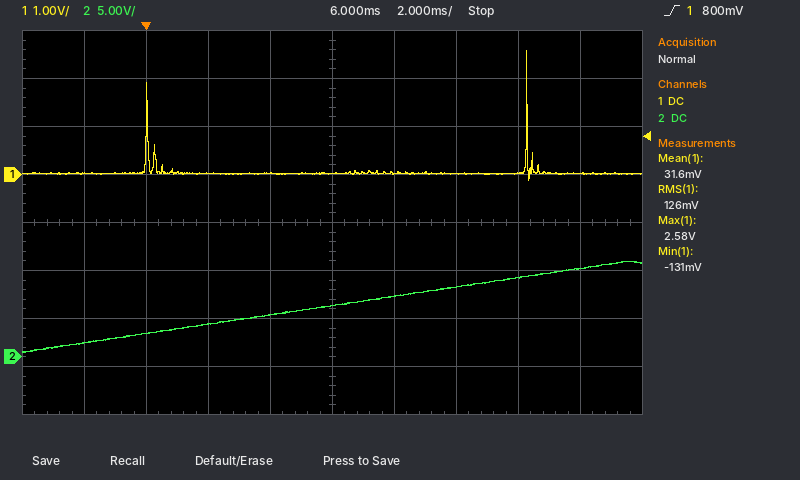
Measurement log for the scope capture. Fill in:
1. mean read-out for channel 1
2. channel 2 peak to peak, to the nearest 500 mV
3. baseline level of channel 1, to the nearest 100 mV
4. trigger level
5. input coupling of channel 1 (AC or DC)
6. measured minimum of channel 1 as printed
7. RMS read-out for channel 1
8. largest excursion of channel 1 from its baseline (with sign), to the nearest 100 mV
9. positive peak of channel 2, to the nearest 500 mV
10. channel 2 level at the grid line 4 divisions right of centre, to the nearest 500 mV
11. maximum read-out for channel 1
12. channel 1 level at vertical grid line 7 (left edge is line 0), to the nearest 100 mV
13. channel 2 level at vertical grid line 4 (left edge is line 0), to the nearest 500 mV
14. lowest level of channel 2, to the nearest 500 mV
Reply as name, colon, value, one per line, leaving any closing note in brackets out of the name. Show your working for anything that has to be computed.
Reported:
mean read-out for channel 1: 31.6 mV
channel 2 peak to peak, to the nearest 500 mV: 10.0 V − (500 mV) = 9.5 V
baseline level of channel 1, to the nearest 100 mV: 0.0 V
trigger level: 800 mV
input coupling of channel 1: DC
measured minimum of channel 1 as printed: -131 mV
RMS read-out for channel 1: 126 mV
largest excursion of channel 1 from its baseline (with sign), to the nearest 100 mV: +2.6 V
positive peak of channel 2, to the nearest 500 mV: 10.0 V
channel 2 level at the grid line 4 divisions right of centre, to the nearest 500 mV: 9.0 V
maximum read-out for channel 1: 2.58 V
channel 1 level at vertical grid line 7 (left edge is line 0), to the nearest 100 mV: 0.0 V
channel 2 level at vertical grid line 4 (left edge is line 0), to the nearest 500 mV: 4.5 V
lowest level of channel 2, to the nearest 500 mV: 500 mV
